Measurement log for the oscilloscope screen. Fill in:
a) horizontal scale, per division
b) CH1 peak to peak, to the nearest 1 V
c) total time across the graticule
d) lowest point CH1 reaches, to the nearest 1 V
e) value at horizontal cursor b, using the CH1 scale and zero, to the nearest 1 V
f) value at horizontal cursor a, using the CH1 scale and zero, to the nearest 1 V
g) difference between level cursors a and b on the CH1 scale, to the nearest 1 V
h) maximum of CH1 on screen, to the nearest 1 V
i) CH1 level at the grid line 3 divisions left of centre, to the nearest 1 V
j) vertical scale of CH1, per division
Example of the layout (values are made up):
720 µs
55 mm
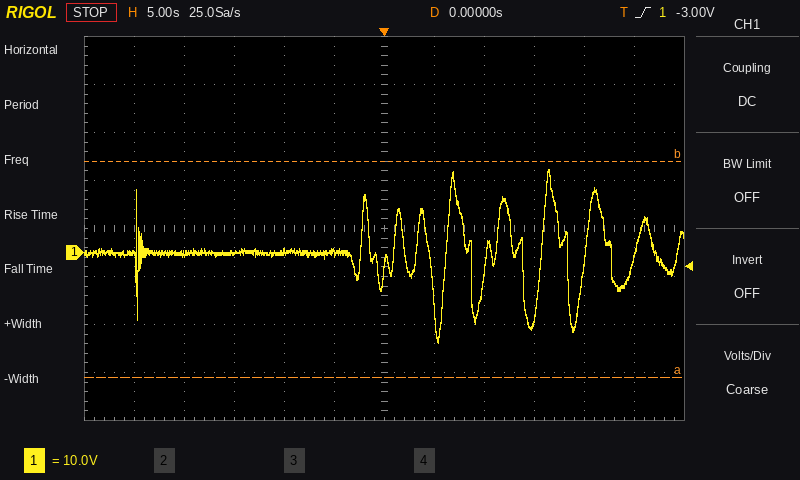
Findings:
5 s
36 V
60 s
-19 V
19 V
-26 V
45 V
17 V
0 V
10 V
